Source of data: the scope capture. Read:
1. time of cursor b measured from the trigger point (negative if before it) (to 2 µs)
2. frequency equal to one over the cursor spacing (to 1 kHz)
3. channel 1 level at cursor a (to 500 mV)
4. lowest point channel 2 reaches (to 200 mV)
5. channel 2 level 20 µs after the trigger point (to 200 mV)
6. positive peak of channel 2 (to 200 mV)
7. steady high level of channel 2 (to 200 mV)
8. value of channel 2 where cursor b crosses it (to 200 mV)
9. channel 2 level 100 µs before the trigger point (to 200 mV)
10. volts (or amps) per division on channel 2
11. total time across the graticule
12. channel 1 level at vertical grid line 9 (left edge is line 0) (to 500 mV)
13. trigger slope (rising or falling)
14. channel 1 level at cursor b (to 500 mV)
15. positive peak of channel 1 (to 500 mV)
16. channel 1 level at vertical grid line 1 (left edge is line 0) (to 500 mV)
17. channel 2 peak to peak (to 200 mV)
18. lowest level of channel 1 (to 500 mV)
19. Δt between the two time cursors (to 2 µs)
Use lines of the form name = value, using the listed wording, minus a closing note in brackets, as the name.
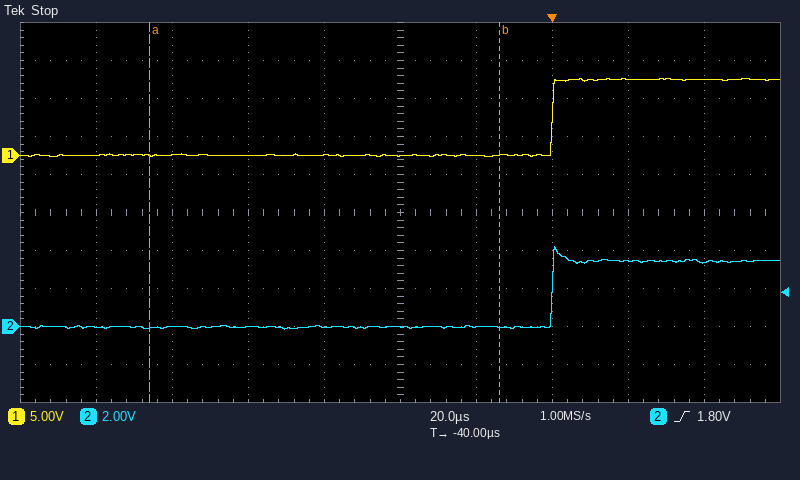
time of cursor b measured from the trigger point (negative if before it) = -14 µs
frequency equal to one over the cursor spacing = 11 kHz
channel 1 level at cursor a = 0.0 V
lowest point channel 2 reaches = -200 mV
channel 2 level 20 µs after the trigger point = 3.4 V
positive peak of channel 2 = 4.2 V
steady high level of channel 2 = 3.4 V
value of channel 2 where cursor b crosses it = 0.0 V
channel 2 level 100 µs before the trigger point = 0.0 V
volts (or amps) per division on channel 2 = 2 V
total time across the graticule = 200 µs
channel 1 level at vertical grid line 9 (left edge is line 0) = 10.0 V
trigger slope = rising
channel 1 level at cursor b = 0.0 V
positive peak of channel 1 = 10.0 V
channel 1 level at vertical grid line 1 (left edge is line 0) = 0.0 V
channel 2 peak to peak = 4.4 V
lowest level of channel 1 = 0.0 V
Δt between the two time cursors = 92 µs
